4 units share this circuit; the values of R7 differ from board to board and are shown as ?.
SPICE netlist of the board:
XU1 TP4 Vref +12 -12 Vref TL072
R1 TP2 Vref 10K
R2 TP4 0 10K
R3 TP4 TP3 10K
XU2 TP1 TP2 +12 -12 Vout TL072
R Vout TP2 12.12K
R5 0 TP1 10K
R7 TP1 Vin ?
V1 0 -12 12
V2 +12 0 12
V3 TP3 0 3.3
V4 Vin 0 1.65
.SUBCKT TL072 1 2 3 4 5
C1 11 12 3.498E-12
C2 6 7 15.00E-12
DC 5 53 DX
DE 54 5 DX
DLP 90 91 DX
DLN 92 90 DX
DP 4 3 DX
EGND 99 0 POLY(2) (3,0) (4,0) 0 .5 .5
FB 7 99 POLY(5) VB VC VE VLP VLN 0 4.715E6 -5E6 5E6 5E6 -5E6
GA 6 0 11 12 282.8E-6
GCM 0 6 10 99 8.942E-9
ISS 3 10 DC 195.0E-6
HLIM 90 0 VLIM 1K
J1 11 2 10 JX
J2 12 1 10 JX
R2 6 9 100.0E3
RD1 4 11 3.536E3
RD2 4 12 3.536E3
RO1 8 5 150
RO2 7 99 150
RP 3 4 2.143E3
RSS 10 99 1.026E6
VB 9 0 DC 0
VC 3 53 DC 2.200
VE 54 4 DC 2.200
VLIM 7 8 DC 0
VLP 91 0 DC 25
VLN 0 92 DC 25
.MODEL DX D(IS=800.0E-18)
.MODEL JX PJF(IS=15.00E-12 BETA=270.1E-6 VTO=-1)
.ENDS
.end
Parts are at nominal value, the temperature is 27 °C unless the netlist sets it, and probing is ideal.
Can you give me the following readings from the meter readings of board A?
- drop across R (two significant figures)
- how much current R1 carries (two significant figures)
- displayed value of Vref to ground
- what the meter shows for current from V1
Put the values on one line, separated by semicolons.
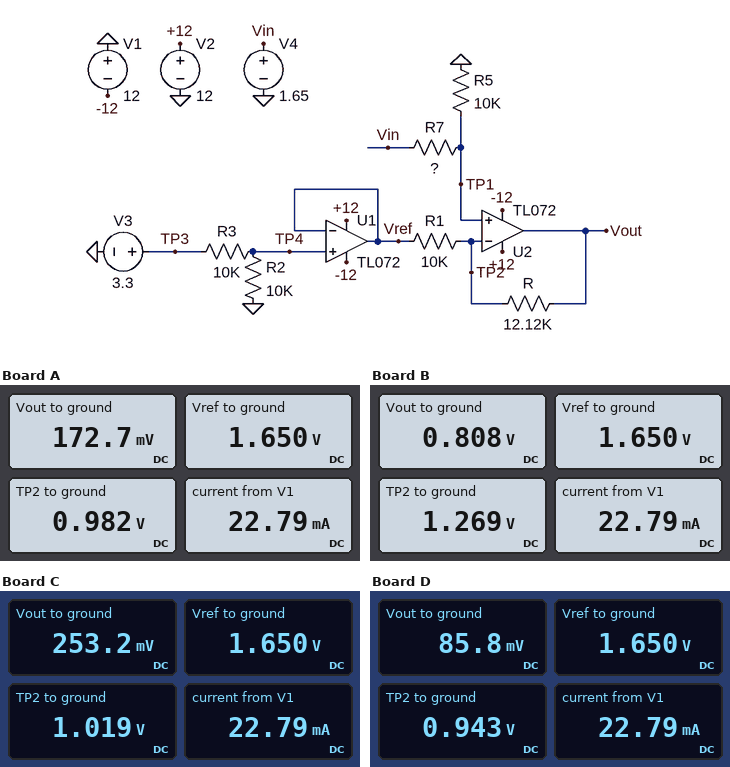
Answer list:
810 mV; 67 µA; 1.650 V; 22.79 mA
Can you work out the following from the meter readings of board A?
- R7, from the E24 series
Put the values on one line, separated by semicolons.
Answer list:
6.8 kΩ
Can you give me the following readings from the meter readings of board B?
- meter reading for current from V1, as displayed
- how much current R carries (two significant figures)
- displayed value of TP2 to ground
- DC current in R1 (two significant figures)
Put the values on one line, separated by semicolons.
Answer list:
22.79 mA; 38 µA; 1.269 V; 38 µA
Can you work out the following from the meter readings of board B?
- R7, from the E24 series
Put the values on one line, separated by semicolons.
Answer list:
3 kΩ
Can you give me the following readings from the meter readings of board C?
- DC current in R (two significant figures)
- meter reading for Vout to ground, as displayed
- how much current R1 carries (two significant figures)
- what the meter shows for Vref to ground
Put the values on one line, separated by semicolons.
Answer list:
63 µA; 253.2 mV; 63 µA; 1.650 V
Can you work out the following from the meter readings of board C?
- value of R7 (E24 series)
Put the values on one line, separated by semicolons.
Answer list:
6.2 kΩ
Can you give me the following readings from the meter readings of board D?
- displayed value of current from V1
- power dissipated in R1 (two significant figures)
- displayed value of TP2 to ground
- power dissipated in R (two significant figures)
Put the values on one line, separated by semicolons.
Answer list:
22.79 mA; 50 µW; 0.943 V; 61 µW
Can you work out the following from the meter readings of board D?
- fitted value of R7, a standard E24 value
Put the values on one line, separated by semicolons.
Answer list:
7.5 kΩ
